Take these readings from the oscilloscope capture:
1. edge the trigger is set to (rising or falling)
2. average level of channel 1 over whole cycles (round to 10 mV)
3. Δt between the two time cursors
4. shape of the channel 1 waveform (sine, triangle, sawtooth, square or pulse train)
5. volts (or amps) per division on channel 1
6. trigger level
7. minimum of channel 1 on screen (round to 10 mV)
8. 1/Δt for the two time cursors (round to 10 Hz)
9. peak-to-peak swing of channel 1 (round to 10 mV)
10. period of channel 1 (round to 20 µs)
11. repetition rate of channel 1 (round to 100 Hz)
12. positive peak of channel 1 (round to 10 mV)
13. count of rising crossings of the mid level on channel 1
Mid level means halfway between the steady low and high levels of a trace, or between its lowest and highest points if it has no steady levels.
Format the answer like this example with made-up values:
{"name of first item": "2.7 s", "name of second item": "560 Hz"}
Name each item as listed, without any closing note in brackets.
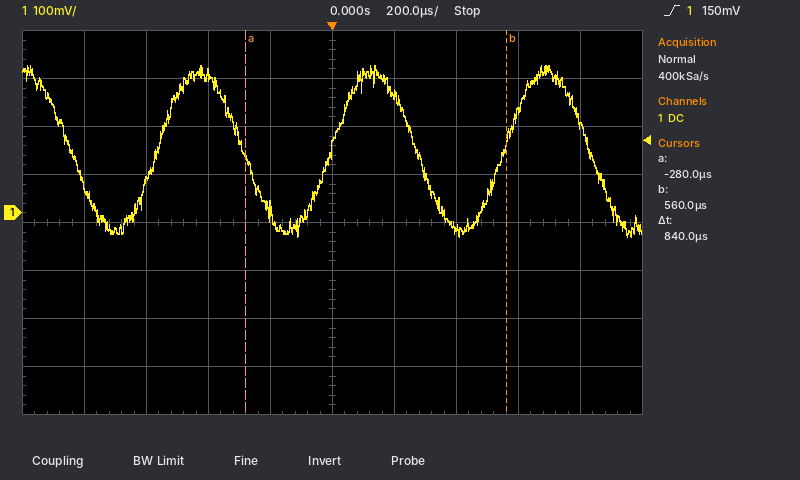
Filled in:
{"edge the trigger is set to": "rising", "average level of channel 1 over whole cycles": "130 mV", "Δt between the two time cursors": "840 µs", "shape of the channel 1 waveform": "sine", "volts (or amps) per division on channel 1": "100 mV", "trigger level": "150 mV", "minimum of channel 1 on screen": "-50 mV", "1/Δt for the two time cursors": "1.19 kHz", "peak-to-peak swing of channel 1": "360 mV", "period of channel 1": "560 µs", "repetition rate of channel 1": "1.8 kHz", "positive peak of channel 1": "310 mV", "count of rising crossings of the mid level on channel 1": "3"}
